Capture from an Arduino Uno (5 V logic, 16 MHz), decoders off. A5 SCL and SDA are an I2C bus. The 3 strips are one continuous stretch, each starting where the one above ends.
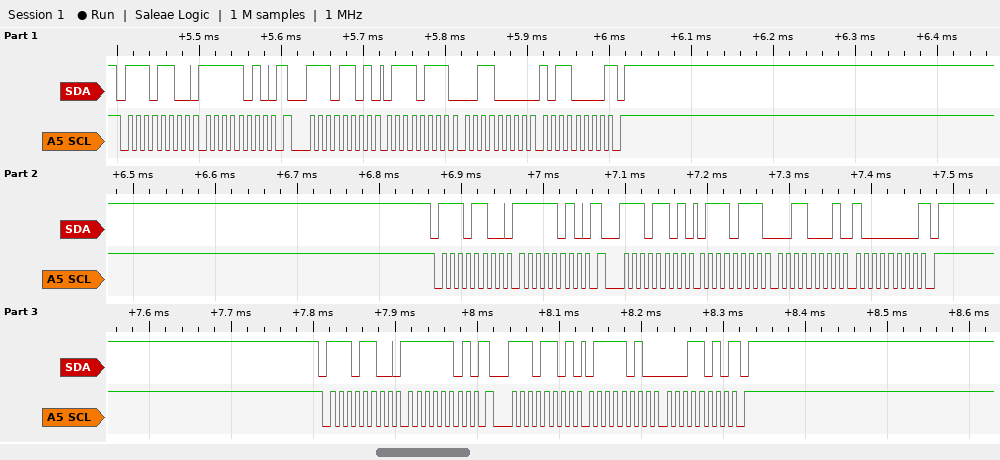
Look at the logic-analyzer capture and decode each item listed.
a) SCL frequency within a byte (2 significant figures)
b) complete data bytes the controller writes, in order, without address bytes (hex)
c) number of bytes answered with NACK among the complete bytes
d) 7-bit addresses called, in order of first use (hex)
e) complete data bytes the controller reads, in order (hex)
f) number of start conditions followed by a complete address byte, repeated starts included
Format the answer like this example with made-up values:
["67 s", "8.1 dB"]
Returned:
["100 kHz", "FA FA FD", "3", "0x76", "77 30 B0 77 31 80 7A 1A", "6"]
